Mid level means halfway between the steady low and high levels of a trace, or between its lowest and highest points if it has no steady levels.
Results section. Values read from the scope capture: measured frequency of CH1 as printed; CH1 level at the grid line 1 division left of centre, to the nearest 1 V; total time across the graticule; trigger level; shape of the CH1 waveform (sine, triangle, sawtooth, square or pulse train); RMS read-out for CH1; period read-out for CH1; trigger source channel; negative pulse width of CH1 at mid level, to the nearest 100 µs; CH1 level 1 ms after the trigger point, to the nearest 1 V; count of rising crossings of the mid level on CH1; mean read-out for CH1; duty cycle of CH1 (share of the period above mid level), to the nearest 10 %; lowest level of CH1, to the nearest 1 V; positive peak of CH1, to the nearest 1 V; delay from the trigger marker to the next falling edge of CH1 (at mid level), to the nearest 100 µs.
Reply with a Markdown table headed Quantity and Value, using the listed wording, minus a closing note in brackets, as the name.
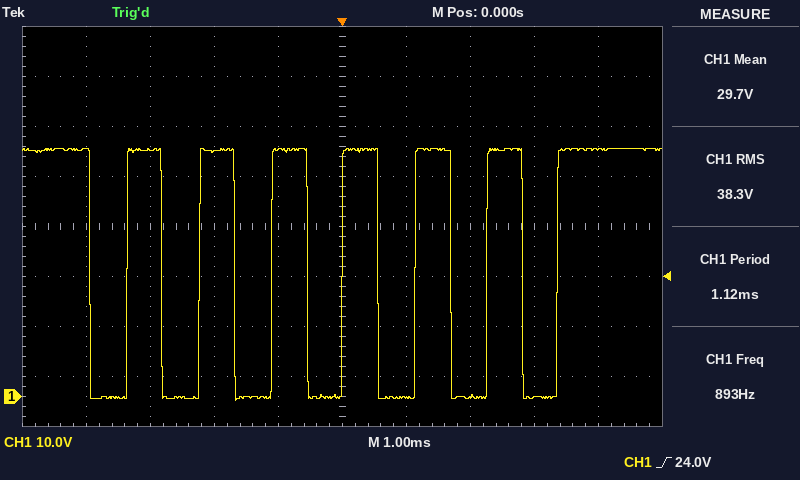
| Quantity | Value |
|---|---|
| measured frequency of CH1 as printed | 893 Hz |
| CH1 level at the grid line 1 division left of centre, to the nearest 1 V | 49 V |
| total time across the graticule | 10 ms |
| trigger level | 24.0 V |
| shape of the CH1 waveform | square |
| RMS read-out for CH1 | 38.3 V |
| period read-out for CH1 | 1.12 ms |
| trigger source channel | CH1 |
| negative pulse width of CH1 at mid level, to the nearest 100 µs | 600 µs |
| CH1 level 1 ms after the trigger point, to the nearest 1 V | 0 V |
| count of rising crossings of the mid level on CH1 | 7 |
| mean read-out for CH1 | 29.7 V |
| duty cycle of CH1 (share of the period above mid level), to the nearest 10 % | 50 % |
| lowest level of CH1, to the nearest 1 V | -1 V |
| positive peak of CH1, to the nearest 1 V | 50 V |
| delay from the trigger marker to the next falling edge of CH1 (at mid level), to the nearest 100 µs | 600 µs |
